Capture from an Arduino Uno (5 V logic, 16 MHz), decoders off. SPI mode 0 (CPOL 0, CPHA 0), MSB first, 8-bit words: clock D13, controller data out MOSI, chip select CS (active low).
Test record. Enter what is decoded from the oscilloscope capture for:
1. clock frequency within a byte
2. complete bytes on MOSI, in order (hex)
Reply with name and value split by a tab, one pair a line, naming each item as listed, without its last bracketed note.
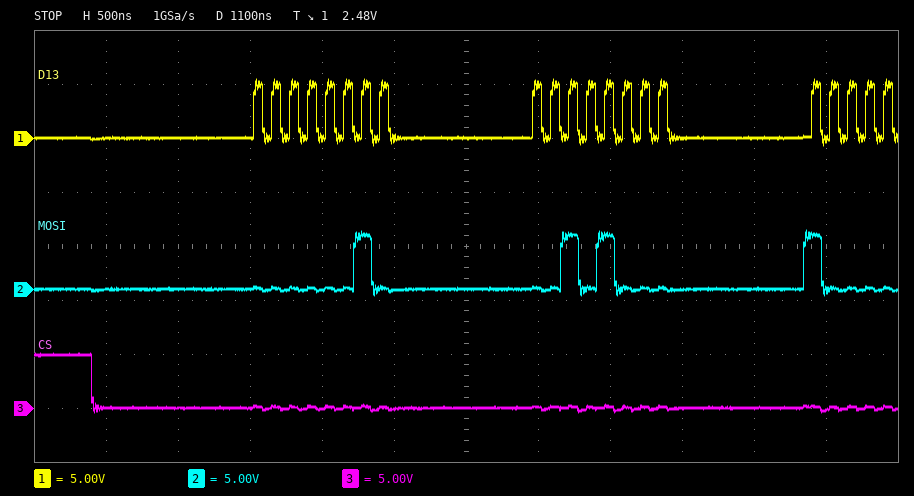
clock frequency within a byte	8 MHz
complete bytes on MOSI, in order	0x02 0x28
